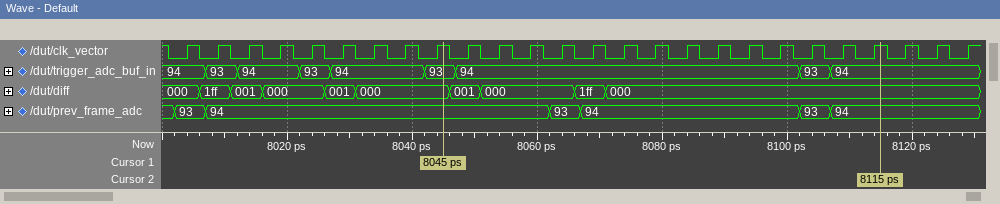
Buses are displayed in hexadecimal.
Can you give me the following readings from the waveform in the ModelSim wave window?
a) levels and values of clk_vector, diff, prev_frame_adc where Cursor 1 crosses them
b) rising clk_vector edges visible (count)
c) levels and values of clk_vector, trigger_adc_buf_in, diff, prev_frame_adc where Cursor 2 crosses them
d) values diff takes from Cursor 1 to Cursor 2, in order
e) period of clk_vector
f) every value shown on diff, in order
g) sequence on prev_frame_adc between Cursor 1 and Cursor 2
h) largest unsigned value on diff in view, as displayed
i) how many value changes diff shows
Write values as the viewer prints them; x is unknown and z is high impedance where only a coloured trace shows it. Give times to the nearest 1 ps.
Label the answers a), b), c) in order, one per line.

a) clk_vector=1, diff=000, prev_frame_adc=94
b) 26
c) clk_vector=1, trigger_adc_buf_in=94, diff=000, prev_frame_adc=94
d) 000, 001, 000, 1ff, 000
e) 5 ps
f) 000, 1ff, 001, 000, 001, 000, 001, 000, 1ff, 000
g) 94, 93, 94, 93, 94
h) 1ff
i) 9
